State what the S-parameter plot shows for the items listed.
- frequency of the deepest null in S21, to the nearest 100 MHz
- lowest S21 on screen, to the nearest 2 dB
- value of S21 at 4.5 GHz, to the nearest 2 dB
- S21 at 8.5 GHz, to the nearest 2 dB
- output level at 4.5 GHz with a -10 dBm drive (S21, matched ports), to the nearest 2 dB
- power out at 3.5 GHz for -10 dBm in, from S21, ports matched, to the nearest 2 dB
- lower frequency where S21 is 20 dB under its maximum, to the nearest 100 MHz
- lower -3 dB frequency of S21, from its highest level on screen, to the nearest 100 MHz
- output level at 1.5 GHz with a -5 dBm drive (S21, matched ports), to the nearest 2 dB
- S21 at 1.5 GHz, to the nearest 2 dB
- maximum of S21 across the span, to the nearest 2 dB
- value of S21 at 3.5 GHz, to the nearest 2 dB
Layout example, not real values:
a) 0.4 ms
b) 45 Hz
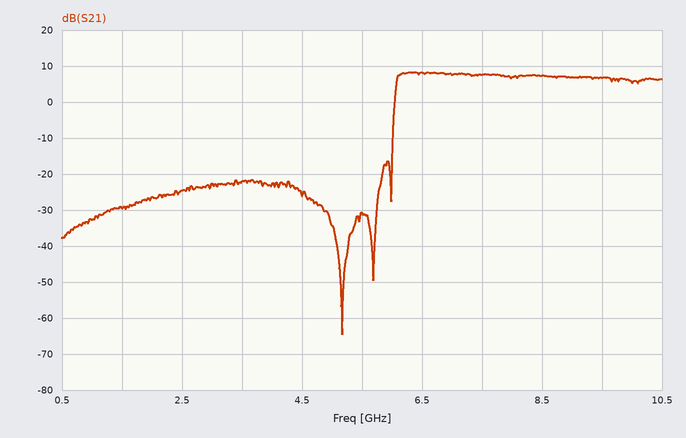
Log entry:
a) 5.2 GHz
b) -64 dB
c) -26 dB
d) 8 dB
e) -36 dBm
f) -32 dBm
g) 6.0 GHz
h) 6.1 GHz
i) -34 dBm
j) -30 dB
k) 8 dB
l) -22 dB
